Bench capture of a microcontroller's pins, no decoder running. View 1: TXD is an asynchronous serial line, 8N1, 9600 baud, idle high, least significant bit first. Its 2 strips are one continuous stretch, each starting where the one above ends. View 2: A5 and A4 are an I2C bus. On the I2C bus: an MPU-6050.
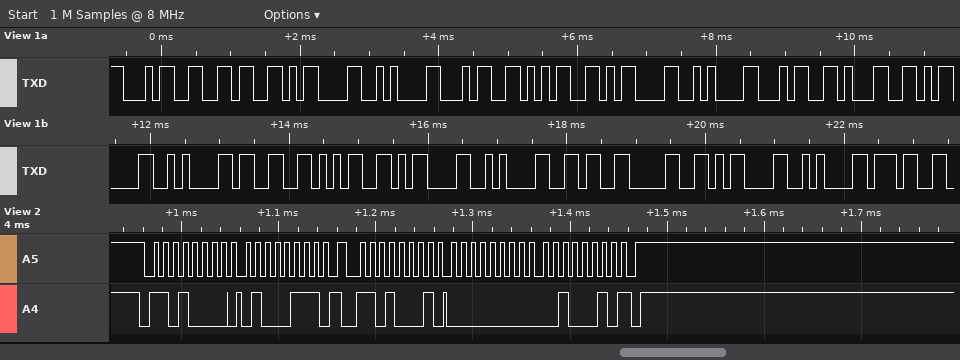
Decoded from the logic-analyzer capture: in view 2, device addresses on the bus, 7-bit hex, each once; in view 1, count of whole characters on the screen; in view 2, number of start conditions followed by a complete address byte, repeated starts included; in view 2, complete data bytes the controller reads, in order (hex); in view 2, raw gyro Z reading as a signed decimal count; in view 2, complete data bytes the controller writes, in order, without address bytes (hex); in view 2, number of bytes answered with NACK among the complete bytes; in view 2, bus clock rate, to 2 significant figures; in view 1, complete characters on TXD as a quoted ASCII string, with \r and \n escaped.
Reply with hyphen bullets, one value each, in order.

- 0x68
- 21
- 2
- 00 22
- 34
- 47
- 1
- 100 kHz
- "46\r\n45\r\n41\r\n35\r\n60\r\n7"
